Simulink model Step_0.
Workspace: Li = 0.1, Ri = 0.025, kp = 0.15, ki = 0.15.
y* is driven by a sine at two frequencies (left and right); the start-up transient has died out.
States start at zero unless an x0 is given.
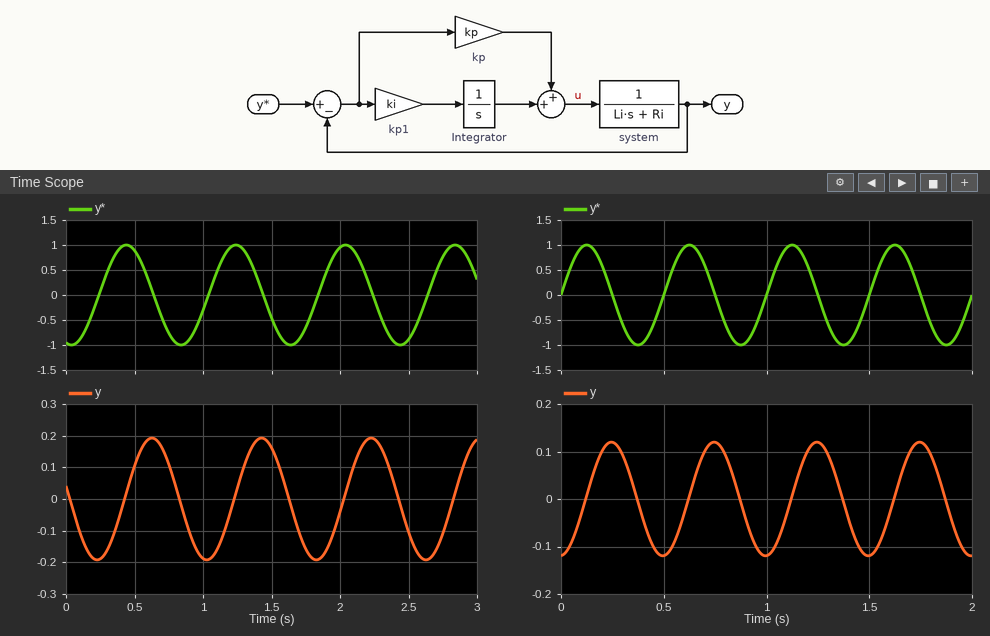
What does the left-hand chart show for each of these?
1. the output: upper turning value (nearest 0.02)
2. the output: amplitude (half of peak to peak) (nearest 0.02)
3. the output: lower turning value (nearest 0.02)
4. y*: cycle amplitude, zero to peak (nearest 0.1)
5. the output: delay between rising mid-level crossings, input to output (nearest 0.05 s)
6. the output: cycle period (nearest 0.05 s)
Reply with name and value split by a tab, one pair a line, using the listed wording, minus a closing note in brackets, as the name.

the output: upper turning value	0.20
the output: amplitude (half of peak to peak)	0.20
the output: lower turning value	-0.20
y*: cycle amplitude, zero to peak	1.0
the output: delay between rising mid-level crossings, input to output	0.20 s
the output: cycle period	0.80 s
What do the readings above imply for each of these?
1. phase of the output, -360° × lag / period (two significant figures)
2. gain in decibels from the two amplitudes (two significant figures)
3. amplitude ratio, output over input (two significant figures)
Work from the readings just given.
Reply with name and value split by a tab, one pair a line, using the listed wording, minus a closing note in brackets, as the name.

phase of the output, -360° × lag / period	-90°
gain in decibels from the two amplitudes	-14 dB
amplitude ratio, output over input	0.20
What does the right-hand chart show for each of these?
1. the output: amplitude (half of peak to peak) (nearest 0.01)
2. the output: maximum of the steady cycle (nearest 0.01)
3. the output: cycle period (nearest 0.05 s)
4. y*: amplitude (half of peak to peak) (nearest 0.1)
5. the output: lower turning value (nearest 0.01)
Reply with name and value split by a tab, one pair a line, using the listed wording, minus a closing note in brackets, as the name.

the output: amplitude (half of peak to peak)	0.12
the output: maximum of the steady cycle	0.12
the output: cycle period	0.50 s
y*: amplitude (half of peak to peak)	1.0
the output: lower turning value	-0.12
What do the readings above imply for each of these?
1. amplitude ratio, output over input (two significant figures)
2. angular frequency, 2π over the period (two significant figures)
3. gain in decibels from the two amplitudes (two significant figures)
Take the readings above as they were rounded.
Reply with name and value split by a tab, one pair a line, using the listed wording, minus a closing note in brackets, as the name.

amplitude ratio, output over input	0.12
angular frequency, 2π over the period	13 rad/s
gain in decibels from the two amplitudes	-18 dB
